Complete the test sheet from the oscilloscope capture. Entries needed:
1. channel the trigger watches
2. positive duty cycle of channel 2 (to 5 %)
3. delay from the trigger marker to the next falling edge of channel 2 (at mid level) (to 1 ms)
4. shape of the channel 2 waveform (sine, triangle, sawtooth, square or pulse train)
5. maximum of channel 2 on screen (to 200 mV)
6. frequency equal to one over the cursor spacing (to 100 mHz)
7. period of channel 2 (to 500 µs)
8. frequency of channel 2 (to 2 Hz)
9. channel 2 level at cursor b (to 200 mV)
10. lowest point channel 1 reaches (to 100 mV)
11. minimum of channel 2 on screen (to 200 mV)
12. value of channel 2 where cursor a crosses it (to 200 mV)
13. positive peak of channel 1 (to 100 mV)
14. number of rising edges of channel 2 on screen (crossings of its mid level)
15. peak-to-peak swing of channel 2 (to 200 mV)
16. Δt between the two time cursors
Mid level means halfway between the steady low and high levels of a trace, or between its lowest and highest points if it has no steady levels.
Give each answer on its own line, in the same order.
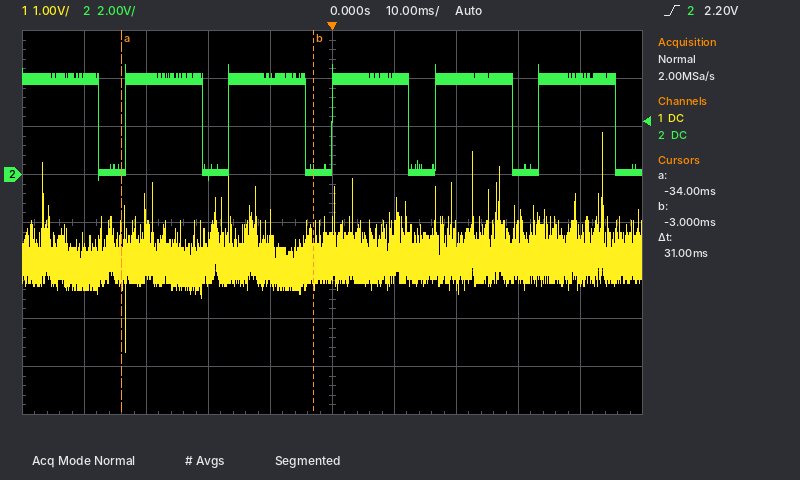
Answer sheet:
channel 2
75 %
12 ms
pulse train
4.6 V
32.3 Hz
16.5 ms
60 Hz
200 mV
-3.7 V
-200 mV
200 mV
900 mV
5
4.8 V
31 ms
